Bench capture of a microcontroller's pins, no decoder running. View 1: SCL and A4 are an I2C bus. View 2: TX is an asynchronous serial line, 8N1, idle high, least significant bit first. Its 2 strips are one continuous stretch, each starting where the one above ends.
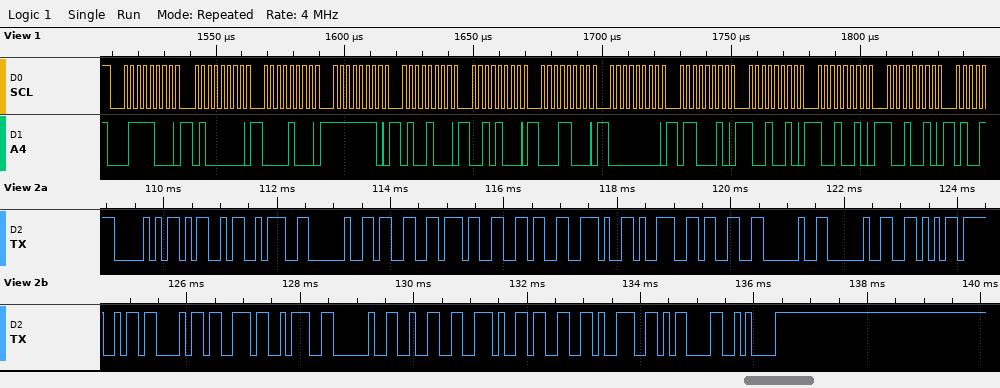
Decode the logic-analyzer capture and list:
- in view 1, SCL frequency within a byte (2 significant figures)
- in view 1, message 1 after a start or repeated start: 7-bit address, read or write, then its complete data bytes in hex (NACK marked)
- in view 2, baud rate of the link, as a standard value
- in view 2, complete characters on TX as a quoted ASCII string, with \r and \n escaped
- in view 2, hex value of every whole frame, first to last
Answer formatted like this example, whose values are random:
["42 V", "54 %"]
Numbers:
["400 kHz", "0x3C write: 40 08 FE 48 28 18 00 62 92 92 92", "9600 baud", "\"PM: 376.93  VOCs: 2.39\\r\\n\"", "50 4D 3A 20 33 37 36 2E 39 33 20 20 56 4F 43 73 3A 20 32 2E 33 39 0D 0A"]
